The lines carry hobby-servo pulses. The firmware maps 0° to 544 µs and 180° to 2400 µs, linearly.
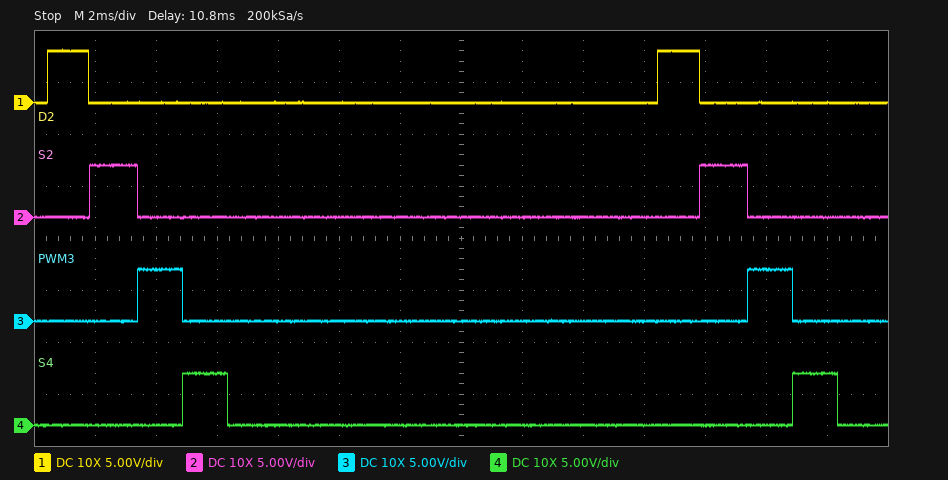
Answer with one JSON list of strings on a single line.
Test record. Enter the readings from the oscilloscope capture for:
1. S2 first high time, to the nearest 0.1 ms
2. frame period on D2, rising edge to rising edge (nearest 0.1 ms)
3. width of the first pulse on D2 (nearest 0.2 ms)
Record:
["1.6 ms", "20.0 ms", "1.4 ms"]
